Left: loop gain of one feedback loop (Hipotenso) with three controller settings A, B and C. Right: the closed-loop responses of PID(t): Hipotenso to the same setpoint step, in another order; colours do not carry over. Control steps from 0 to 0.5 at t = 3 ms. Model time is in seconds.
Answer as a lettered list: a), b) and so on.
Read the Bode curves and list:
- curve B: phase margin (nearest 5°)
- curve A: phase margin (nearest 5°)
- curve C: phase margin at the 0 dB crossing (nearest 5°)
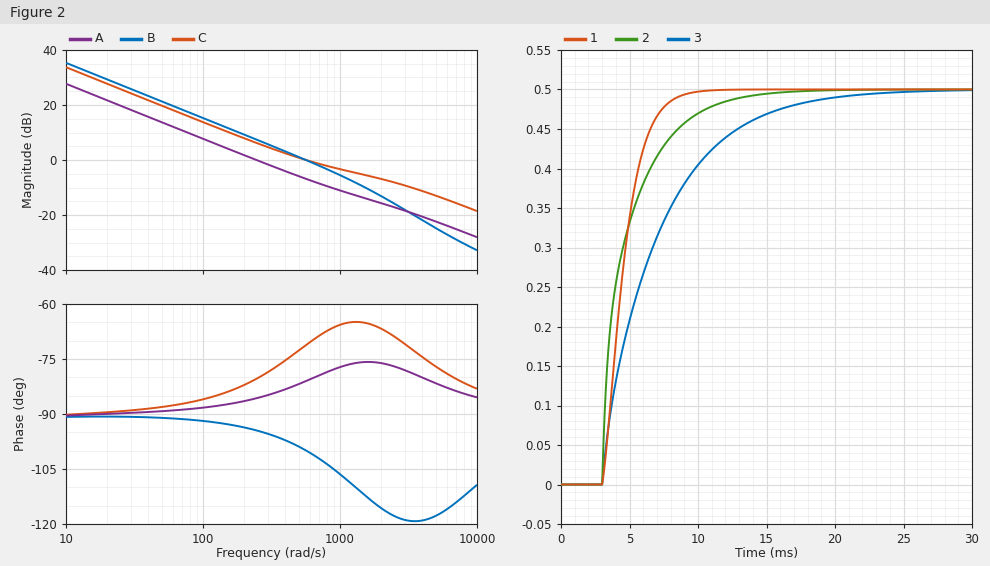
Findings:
a) 80°
b) 95°
c) 110°
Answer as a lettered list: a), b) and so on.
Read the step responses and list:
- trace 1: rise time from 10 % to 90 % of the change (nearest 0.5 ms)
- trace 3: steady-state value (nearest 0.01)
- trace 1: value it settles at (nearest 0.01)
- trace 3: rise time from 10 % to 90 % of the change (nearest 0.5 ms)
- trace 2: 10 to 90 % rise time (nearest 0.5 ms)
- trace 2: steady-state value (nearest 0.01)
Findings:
a) 3.0 ms
b) 0.50
c) 0.50
d) 9.5 ms
e) 5.5 ms
f) 0.50
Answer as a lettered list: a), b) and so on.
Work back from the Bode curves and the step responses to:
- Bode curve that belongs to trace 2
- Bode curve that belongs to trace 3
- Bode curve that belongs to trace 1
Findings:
a) C
b) A
c) B
